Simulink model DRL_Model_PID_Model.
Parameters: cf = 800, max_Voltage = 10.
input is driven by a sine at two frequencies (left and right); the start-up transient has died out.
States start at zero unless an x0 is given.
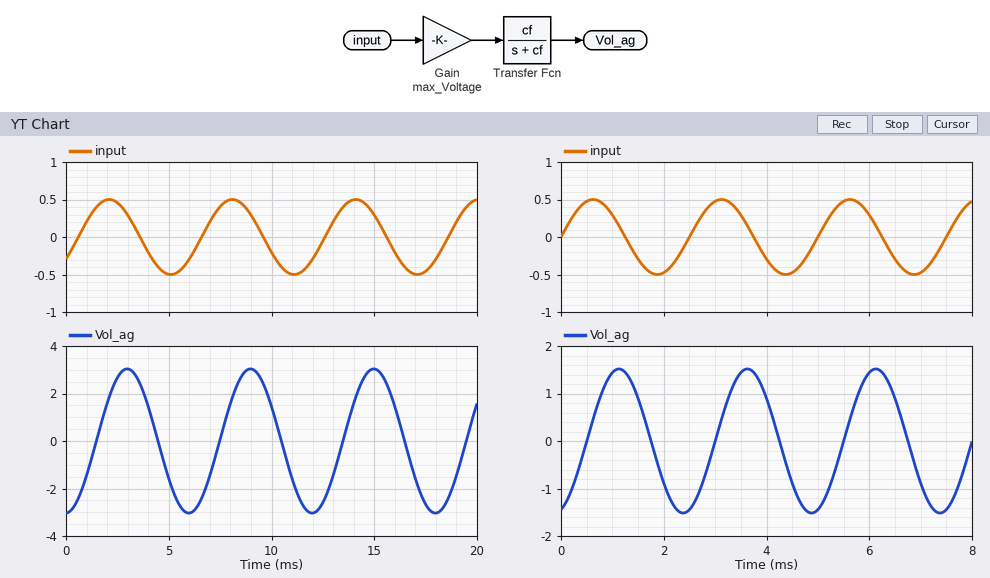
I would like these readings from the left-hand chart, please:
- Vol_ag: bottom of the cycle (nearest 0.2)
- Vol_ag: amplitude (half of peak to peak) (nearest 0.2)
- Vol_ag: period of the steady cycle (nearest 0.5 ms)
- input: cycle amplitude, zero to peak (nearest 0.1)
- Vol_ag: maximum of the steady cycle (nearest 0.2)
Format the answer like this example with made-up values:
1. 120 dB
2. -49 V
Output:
1. -3.0
2. 3.0
3. 6.0 ms
4. 0.5
5. 3.0
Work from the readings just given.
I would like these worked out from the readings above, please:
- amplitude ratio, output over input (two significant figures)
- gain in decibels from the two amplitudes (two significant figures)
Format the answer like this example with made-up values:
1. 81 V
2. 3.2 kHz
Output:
1. 6.0
2. 16 dB
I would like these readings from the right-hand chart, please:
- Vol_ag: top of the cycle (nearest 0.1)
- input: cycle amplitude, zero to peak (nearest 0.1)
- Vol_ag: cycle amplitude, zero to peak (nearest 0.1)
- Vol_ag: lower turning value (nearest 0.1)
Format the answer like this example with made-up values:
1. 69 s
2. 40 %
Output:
1. 1.5
2. 0.5
3. 1.5
4. -1.5
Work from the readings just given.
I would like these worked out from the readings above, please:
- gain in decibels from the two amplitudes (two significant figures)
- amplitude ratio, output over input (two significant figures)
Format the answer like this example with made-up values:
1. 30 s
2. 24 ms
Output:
1. 9.5 dB
2. 3.0
